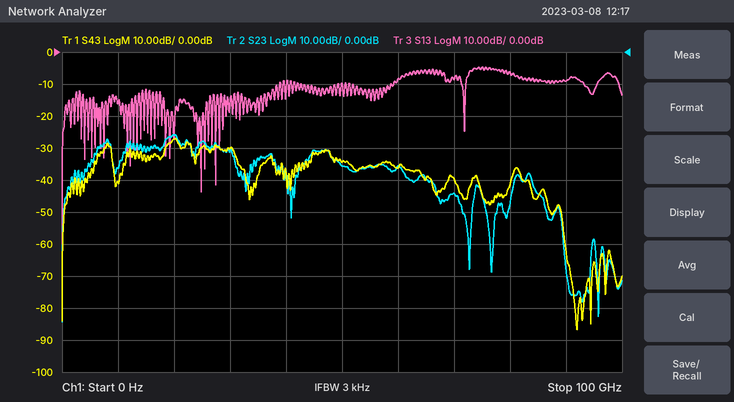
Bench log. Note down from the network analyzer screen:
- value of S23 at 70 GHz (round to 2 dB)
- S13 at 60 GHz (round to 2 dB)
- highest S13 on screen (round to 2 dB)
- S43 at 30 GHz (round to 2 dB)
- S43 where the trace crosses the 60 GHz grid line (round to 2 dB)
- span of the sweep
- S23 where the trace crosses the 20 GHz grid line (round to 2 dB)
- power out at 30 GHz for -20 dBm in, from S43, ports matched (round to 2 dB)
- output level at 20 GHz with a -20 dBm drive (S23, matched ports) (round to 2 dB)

-44 dB
-8 dB
-4 dB
-30 dB
-36 dB
100 GHz
-26 dB
-50 dBm
-46 dBm
